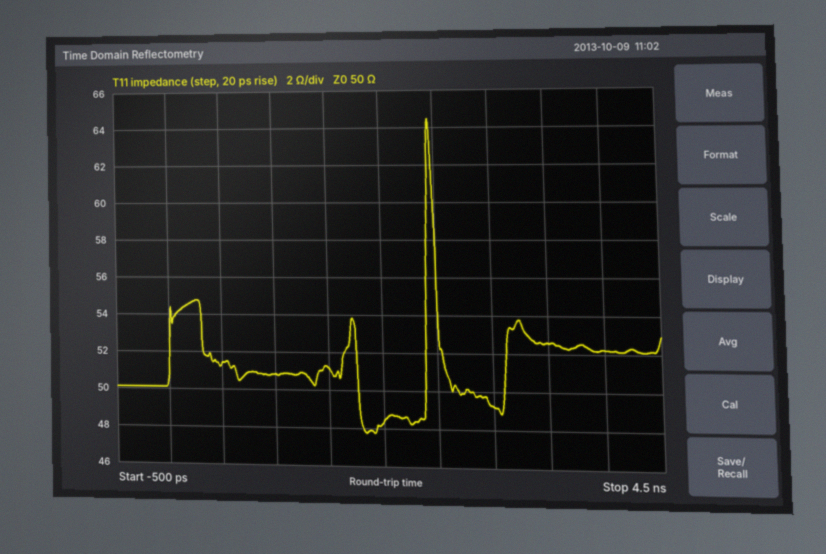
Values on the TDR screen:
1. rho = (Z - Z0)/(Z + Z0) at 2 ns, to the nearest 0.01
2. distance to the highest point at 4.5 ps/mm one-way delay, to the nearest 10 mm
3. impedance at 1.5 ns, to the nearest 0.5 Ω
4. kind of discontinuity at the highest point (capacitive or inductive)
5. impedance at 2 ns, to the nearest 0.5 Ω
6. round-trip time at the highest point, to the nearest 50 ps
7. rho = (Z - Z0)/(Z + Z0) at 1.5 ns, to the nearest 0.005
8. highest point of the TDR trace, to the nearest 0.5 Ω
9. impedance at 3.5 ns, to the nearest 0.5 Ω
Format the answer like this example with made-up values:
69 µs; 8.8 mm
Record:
-0.02; 270 mm; 51.0 Ω; inductive; 48.5 Ω; 2.45 ns; +0.010; 64.5 Ω; 52.5 Ω
